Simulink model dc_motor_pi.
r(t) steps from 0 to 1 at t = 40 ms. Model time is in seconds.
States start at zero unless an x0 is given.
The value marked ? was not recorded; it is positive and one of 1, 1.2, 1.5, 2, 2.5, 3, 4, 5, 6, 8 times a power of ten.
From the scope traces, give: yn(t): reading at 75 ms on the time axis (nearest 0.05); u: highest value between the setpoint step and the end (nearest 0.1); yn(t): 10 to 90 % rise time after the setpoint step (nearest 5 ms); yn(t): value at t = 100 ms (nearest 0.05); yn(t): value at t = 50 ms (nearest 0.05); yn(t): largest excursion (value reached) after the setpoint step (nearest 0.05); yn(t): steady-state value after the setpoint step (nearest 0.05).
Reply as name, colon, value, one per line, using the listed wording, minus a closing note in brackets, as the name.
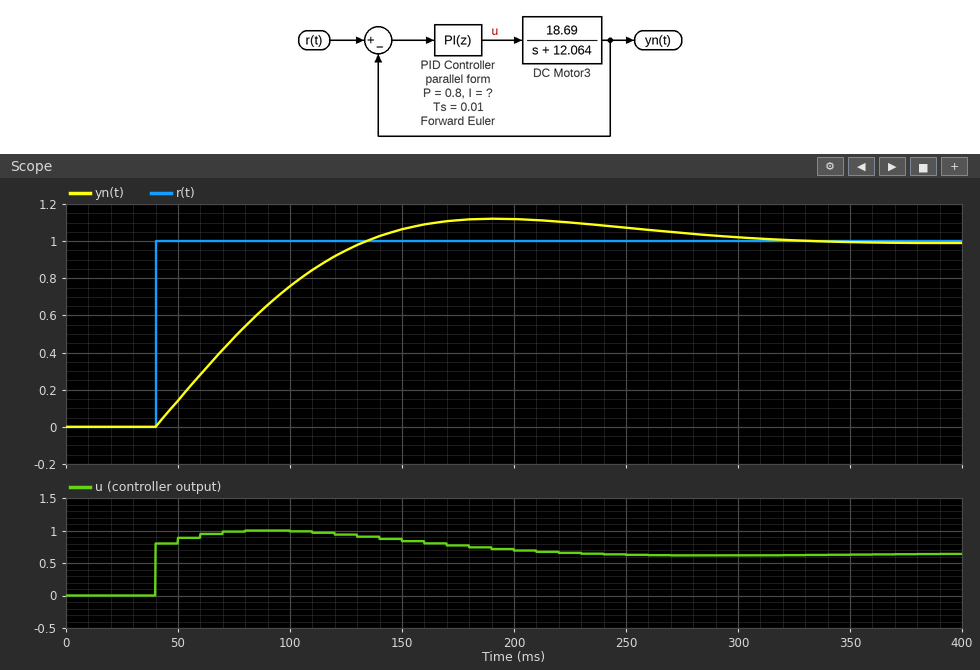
yn(t): reading at 75 ms on the time axis: 0.50
u: highest value between the setpoint step and the end: 1.0
yn(t): 10 to 90 % rise time after the setpoint step: 70 ms
yn(t): value at t = 100 ms: 0.75
yn(t): value at t = 50 ms: 0.15
yn(t): largest excursion (value reached) after the setpoint step: 1.10
yn(t): steady-state value after the setpoint step: 1.00
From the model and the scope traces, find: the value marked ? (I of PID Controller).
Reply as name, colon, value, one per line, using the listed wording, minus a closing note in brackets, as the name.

the value marked ?: 20
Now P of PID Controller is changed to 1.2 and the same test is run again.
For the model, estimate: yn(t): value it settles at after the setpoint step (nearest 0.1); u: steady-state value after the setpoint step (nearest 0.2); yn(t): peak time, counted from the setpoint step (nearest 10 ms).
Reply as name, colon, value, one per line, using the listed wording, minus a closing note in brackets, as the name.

yn(t): value it settles at after the setpoint step: 1.0
u: steady-state value after the setpoint step: 0.6
yn(t): peak time, counted from the setpoint step: 150 ms
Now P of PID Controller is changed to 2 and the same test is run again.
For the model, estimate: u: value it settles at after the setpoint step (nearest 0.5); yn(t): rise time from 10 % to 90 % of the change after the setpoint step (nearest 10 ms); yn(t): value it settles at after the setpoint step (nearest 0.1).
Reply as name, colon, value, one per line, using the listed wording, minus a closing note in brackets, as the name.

u: value it settles at after the setpoint step: 0.5
yn(t): rise time from 10 % to 90 % of the change after the setpoint step: 60 ms
yn(t): value it settles at after the setpoint step: 1.0
